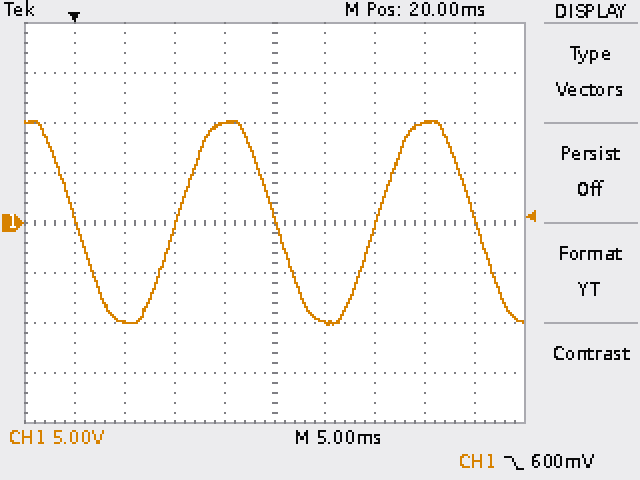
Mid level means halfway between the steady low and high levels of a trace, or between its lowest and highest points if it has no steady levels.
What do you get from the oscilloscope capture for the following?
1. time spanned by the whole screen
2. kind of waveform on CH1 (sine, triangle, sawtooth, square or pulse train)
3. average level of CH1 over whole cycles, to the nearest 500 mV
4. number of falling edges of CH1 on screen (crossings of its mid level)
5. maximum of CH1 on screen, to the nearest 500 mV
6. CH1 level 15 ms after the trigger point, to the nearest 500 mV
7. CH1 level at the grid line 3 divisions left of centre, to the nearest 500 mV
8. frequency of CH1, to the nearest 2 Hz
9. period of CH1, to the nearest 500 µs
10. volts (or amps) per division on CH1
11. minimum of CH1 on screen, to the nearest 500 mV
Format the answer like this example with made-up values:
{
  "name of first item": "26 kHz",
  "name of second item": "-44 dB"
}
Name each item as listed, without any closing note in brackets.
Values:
{
  "time spanned by the whole screen": "50 ms",
  "kind of waveform on CH1": "sine",
  "average level of CH1 over whole cycles, to the nearest 500 mV": "0.0 V",
  "number of falling edges of CH1 on screen": "3",
  "maximum of CH1 on screen, to the nearest 500 mV": "10.0 V",
  "CH1 level 15 ms after the trigger point, to the nearest 500 mV": "10.0 V",
  "CH1 level at the grid line 3 divisions left of centre, to the nearest 500 mV": "-10.0 V",
  "frequency of CH1, to the nearest 2 Hz": "50 Hz",
  "period of CH1, to the nearest 500 µs": "20.0 ms",
  "volts (or amps) per division on CH1": "5 V",
  "minimum of CH1 on screen, to the nearest 500 mV": "-10.0 V"
}
